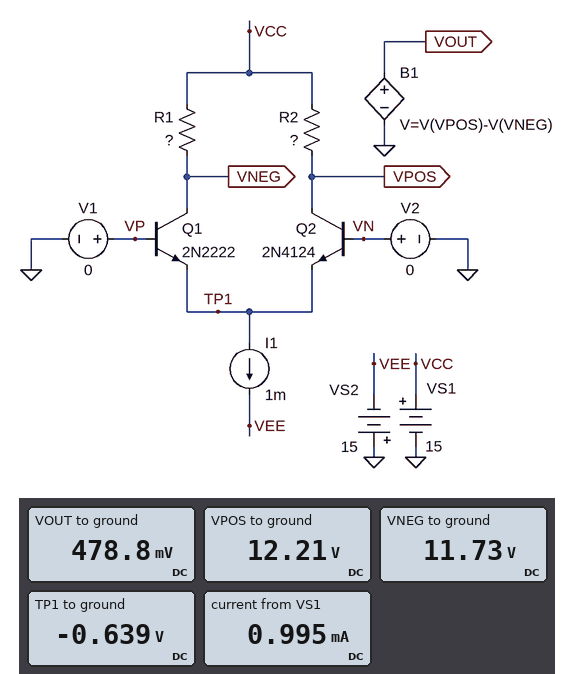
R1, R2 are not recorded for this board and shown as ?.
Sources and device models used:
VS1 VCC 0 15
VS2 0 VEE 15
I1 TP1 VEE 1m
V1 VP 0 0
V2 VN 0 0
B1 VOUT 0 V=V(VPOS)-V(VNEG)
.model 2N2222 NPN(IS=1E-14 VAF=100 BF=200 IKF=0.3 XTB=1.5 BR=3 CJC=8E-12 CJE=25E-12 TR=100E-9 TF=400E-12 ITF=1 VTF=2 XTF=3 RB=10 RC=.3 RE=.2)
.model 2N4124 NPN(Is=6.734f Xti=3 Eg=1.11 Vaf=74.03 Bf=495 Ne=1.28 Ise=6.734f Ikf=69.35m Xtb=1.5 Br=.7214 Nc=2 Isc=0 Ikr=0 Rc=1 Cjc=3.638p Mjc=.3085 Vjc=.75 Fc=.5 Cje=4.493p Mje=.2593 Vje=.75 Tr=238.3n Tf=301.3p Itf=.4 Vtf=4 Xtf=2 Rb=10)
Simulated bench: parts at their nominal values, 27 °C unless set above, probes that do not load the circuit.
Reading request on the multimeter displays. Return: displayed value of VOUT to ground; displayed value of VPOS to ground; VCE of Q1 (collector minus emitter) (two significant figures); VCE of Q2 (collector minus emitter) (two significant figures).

478.8 mV
12.21 V
12 V
13 V
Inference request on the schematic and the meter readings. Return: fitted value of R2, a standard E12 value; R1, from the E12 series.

6.8 kΩ
5.6 kΩ
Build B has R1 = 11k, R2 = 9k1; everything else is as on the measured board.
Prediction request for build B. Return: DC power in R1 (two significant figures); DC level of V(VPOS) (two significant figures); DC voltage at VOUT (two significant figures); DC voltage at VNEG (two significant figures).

3.7 mW
11 V
2.6 V
8.6 V
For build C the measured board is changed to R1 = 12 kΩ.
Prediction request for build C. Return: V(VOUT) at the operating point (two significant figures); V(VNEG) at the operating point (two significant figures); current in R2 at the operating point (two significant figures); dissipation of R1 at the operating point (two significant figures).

4.1 V
8.1 V
420 µA
4.0 mW
